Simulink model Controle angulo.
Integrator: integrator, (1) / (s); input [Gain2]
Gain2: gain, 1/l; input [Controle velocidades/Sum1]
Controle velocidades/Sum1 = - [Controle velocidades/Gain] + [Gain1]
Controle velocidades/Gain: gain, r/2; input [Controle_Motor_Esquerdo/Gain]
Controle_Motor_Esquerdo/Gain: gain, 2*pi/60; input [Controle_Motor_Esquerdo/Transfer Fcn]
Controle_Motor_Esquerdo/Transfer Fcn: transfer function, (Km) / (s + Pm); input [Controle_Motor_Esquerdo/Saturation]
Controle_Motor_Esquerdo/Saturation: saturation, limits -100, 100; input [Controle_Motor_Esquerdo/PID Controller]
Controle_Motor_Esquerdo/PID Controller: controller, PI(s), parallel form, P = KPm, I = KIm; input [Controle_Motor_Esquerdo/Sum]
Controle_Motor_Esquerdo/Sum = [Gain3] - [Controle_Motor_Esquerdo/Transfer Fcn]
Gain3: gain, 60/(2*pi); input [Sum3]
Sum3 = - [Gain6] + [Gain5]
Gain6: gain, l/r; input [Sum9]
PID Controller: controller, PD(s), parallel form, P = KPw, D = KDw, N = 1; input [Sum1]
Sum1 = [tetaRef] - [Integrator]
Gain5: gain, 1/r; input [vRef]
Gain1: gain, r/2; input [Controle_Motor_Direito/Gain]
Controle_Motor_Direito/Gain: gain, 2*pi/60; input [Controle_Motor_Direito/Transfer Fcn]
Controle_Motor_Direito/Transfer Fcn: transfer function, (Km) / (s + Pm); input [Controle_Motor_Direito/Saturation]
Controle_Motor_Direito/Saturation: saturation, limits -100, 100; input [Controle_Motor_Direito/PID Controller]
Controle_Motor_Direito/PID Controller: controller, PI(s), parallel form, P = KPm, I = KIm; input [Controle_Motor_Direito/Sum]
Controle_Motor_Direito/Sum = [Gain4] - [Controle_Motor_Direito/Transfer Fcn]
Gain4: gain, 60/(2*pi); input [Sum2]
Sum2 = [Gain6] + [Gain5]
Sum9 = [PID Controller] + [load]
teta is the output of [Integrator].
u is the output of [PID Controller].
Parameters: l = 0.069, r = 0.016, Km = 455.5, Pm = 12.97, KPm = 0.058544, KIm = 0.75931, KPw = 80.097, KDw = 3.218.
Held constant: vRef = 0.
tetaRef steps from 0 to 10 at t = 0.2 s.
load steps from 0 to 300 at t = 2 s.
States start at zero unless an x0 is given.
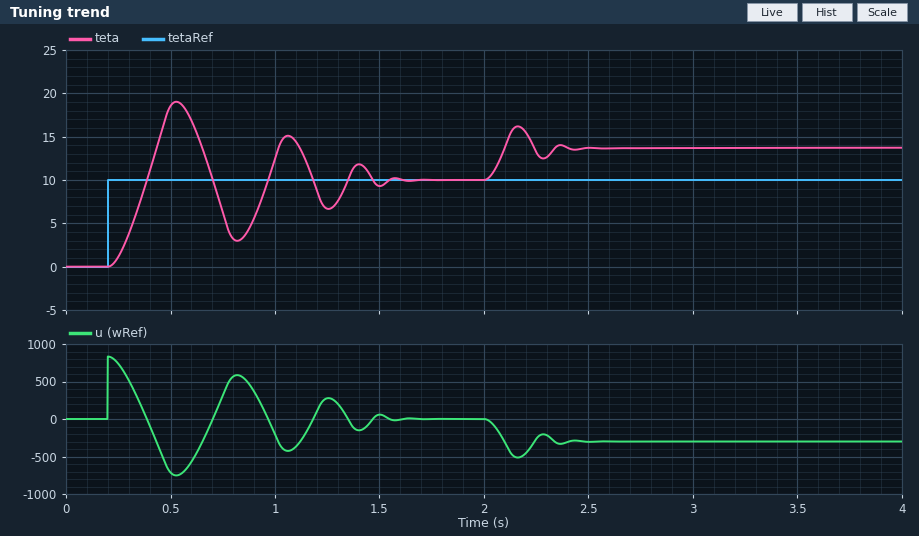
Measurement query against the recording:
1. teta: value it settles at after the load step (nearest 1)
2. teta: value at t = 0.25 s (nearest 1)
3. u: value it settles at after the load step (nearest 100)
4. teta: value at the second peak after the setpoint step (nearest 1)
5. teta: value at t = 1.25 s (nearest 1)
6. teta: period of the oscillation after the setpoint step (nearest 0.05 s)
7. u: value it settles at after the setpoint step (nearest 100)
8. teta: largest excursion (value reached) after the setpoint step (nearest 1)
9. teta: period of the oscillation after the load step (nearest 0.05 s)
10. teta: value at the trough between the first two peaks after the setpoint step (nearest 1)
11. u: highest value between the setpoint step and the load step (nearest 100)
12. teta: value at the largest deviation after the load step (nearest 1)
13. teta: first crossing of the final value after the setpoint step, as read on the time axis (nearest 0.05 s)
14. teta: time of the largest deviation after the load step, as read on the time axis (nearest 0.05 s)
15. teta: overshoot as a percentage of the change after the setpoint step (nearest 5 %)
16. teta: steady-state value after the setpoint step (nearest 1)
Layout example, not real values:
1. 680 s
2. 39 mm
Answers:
1. 14
2. 1
3. -300
4. 15
5. 7
6. 0.55 s
7. 0
8. 19
9. 0.20 s
10. 3
11. 800
12. 16
13. 0.40 s
14. 2.15 s
15. 90 %
16. 10
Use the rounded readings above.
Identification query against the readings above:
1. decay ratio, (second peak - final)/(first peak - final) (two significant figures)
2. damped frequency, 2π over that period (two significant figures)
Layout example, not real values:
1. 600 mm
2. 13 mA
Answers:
1. 0.56
2. 11 rad/s
